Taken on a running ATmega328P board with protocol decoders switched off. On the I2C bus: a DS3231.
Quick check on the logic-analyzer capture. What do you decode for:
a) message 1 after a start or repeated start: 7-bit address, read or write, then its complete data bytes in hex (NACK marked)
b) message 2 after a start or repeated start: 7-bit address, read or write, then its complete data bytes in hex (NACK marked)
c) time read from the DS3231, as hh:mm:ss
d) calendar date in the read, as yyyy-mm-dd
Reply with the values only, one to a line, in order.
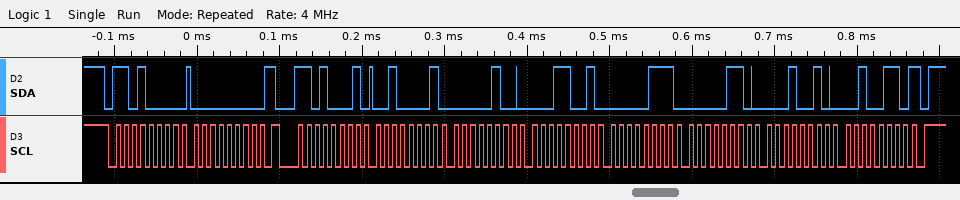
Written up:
0x68 write: 00
0x68 read: 21 04 19 07 06 12 26 NACK
19:04:21
2026-12-06
